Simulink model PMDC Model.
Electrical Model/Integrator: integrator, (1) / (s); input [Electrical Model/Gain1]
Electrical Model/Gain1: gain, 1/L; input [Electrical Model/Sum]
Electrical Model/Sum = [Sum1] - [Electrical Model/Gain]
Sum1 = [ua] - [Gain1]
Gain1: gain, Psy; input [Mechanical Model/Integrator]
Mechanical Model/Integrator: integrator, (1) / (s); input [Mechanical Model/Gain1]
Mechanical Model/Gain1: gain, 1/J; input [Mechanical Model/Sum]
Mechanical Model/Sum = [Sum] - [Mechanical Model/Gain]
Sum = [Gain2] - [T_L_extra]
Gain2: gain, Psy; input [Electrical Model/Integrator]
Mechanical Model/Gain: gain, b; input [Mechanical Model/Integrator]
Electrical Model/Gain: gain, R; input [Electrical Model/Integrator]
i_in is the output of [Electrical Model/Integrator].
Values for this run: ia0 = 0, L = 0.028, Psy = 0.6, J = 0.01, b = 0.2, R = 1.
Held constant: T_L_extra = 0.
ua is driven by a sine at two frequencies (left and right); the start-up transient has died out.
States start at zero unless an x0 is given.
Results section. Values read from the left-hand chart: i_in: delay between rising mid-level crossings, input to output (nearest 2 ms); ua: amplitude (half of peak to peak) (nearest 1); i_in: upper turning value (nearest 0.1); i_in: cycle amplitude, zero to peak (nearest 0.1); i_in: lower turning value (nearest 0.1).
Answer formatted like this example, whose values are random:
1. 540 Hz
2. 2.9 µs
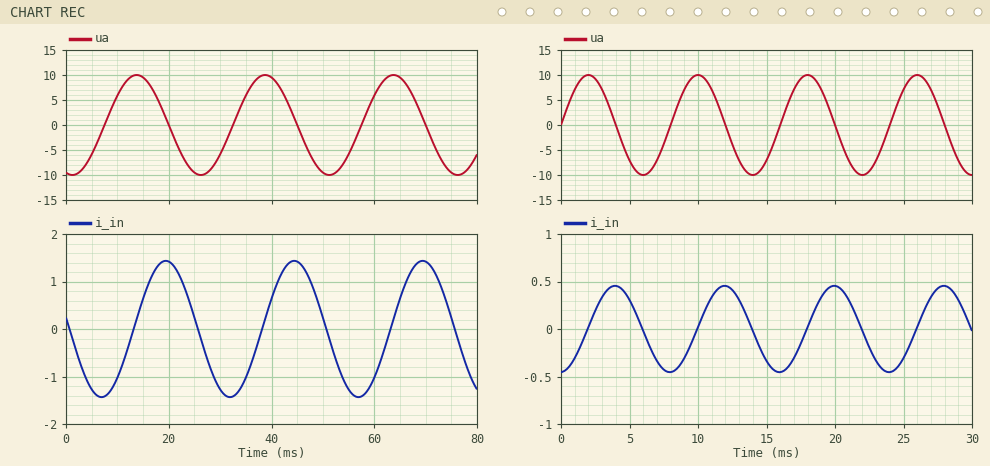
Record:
1. 6 ms
2. 10
3. 1.4
4. 1.4
5. -1.4
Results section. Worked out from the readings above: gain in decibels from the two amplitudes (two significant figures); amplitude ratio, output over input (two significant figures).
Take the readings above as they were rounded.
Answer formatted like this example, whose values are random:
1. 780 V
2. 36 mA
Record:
1. -17 dB
2. 0.14
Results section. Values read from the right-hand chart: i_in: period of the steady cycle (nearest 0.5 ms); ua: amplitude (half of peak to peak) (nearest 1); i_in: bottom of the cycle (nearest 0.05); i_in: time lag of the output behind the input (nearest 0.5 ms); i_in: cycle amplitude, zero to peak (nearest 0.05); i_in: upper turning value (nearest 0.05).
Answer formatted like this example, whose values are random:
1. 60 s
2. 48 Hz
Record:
1. 8.0 ms
2. 10
3. -0.45
4. 2.0 ms
5. 0.45
6. 0.45
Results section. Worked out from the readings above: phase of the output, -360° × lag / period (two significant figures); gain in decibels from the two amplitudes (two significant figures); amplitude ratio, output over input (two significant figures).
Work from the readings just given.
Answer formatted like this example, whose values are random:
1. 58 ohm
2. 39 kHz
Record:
1. -90°
2. -27 dB
3. 0.045
